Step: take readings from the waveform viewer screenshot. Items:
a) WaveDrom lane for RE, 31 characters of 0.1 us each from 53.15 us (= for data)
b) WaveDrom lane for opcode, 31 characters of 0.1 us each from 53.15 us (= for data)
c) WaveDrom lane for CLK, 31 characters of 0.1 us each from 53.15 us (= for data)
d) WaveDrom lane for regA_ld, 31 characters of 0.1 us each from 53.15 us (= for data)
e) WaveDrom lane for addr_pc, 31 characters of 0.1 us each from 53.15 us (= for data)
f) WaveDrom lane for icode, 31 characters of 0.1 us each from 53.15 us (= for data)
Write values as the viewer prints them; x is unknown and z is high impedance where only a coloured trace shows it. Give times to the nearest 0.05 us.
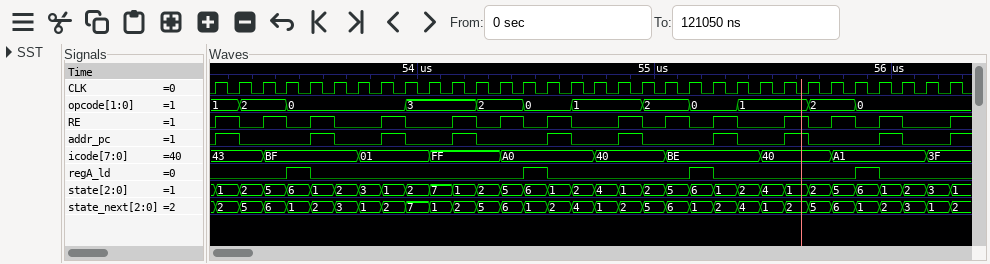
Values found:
{name: 'RE', wave: '101010.10.101010.101010.101010.'}
{name: 'opcode', wave: '==.=....=..=.=.=..=.=.=..=.=...', data: '1 2 0 3 2 0 1 2 0 1 2 0'}
{name: 'CLK', wave: 'p..............................'}
{name: 'regA_ld', wave: '0..10........10.....10.....10..'}
{name: 'addr_pc', wave: '10..10.10.10..10.10..10.10..10.'}
{name: 'icode', wave: '=.=...=..=..=...=..=...=..=...=', data: '43 BF 01 FF A0 40 BE 40 A1 3F'}
